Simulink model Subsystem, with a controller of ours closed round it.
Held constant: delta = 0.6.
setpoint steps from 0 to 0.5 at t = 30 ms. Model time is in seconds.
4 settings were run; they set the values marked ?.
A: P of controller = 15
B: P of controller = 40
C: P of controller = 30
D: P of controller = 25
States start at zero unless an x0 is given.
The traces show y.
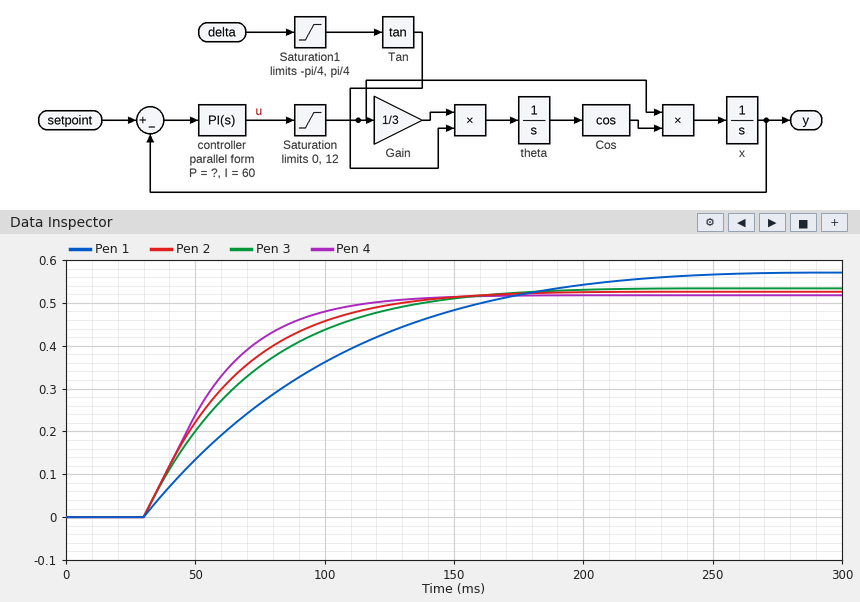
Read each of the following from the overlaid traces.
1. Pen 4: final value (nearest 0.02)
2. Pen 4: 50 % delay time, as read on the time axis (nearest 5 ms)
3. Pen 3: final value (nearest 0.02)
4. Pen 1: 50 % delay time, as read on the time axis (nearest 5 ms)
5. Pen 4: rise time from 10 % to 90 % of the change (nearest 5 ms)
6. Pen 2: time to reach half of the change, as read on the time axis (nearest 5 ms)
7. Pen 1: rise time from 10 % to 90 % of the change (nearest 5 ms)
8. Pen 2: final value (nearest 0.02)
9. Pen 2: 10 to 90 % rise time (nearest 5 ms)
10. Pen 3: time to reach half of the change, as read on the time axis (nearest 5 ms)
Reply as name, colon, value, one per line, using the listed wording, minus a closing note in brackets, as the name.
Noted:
Pen 4: final value: 0.52
Pen 4: 50 % delay time, as read on the time axis: 50 ms
Pen 3: final value: 0.54
Pen 1: 50 % delay time, as read on the time axis: 80 ms
Pen 4: rise time from 10 % to 90 % of the change: 60 ms
Pen 2: time to reach half of the change, as read on the time axis: 55 ms
Pen 1: rise time from 10 % to 90 % of the change: 135 ms
Pen 2: final value: 0.52
Pen 2: 10 to 90 % rise time: 75 ms
Pen 3: time to reach half of the change, as read on the time axis: 60 ms
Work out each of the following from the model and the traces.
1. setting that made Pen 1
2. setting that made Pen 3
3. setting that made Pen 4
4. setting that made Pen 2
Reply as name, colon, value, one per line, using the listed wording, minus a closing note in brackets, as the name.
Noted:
setting that made Pen 1: A
setting that made Pen 3: D
setting that made Pen 4: B
setting that made Pen 2: C
